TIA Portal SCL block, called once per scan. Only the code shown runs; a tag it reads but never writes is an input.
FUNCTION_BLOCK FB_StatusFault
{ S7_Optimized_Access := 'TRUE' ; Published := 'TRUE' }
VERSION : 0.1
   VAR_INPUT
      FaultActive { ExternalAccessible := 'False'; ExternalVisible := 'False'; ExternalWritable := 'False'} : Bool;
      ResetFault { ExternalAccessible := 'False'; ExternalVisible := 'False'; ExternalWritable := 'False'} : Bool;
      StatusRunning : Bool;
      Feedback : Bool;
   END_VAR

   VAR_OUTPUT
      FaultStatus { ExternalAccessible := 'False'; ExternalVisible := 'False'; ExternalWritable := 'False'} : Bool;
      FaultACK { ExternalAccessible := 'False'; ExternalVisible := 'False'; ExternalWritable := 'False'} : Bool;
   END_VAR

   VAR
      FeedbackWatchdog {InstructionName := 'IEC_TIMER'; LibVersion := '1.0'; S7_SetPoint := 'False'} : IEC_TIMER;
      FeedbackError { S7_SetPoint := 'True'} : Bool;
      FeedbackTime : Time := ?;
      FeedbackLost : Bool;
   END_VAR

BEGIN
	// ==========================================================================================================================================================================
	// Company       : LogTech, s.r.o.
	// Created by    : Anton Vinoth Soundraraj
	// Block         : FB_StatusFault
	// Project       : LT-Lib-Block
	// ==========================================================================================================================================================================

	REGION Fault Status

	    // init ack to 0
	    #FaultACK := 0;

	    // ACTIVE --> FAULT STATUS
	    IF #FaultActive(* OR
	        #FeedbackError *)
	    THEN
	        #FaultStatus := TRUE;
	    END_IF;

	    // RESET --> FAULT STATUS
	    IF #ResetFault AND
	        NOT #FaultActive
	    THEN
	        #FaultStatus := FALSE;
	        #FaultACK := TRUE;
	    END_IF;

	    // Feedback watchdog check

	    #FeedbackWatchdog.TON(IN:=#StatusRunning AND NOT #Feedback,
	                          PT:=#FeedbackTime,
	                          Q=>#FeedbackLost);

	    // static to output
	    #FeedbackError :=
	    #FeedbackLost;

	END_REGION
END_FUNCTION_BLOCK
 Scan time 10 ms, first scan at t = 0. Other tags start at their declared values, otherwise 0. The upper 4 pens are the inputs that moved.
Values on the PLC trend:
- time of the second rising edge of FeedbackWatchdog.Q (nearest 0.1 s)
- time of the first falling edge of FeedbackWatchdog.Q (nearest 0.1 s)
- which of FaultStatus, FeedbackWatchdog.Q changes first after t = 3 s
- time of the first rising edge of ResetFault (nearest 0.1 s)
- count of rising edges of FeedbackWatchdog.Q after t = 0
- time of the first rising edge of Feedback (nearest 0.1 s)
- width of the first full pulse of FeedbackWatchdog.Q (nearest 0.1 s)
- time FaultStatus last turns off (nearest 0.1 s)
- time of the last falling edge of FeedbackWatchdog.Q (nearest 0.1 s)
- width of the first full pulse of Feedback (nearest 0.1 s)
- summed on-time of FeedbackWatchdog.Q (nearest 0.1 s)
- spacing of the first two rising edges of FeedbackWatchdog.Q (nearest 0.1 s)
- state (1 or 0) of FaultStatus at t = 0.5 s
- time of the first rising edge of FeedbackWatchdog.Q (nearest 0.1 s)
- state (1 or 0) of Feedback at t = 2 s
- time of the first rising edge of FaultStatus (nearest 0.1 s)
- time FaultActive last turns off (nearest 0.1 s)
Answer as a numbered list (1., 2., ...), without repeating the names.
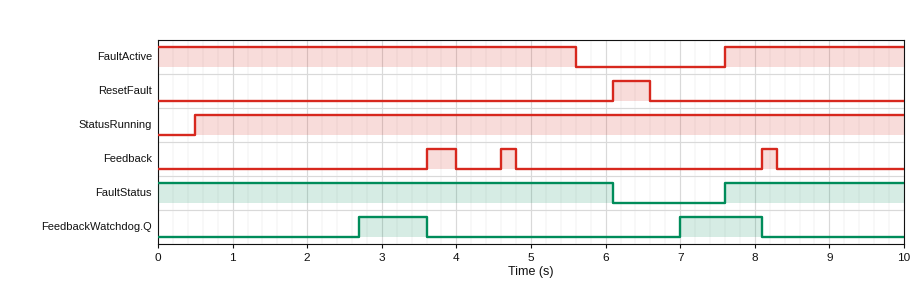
1. 7.0 s
2. 3.6 s
3. FeedbackWatchdog.Q
4. 6.1 s
5. 2
6. 3.6 s
7. 0.9 s
8. 6.1 s
9. 8.1 s
10. 0.4 s
11. 2.0 s
12. 4.3 s
13. 1
14. 2.7 s
15. 0
16. 7.6 s
17. 5.6 s
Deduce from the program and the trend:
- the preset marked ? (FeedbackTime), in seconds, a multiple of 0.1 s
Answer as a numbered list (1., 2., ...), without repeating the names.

1. 2.2 s
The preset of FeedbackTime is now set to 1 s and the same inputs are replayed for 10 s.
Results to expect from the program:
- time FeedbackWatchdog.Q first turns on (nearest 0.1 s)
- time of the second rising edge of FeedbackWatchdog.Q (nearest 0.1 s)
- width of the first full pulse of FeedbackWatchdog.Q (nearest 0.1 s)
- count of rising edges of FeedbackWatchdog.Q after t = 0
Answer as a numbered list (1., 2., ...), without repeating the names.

1. 1.5 s
2. 5.8 s
3. 2.1 s
4. 3
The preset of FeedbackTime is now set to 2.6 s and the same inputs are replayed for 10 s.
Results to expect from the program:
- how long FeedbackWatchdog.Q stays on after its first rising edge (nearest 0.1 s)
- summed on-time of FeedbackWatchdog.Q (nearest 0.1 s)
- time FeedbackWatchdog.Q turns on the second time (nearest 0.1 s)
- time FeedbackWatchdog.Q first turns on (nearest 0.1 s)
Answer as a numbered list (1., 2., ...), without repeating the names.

1. 0.5 s
2. 1.2 s
3. 7.4 s
4. 3.1 s
